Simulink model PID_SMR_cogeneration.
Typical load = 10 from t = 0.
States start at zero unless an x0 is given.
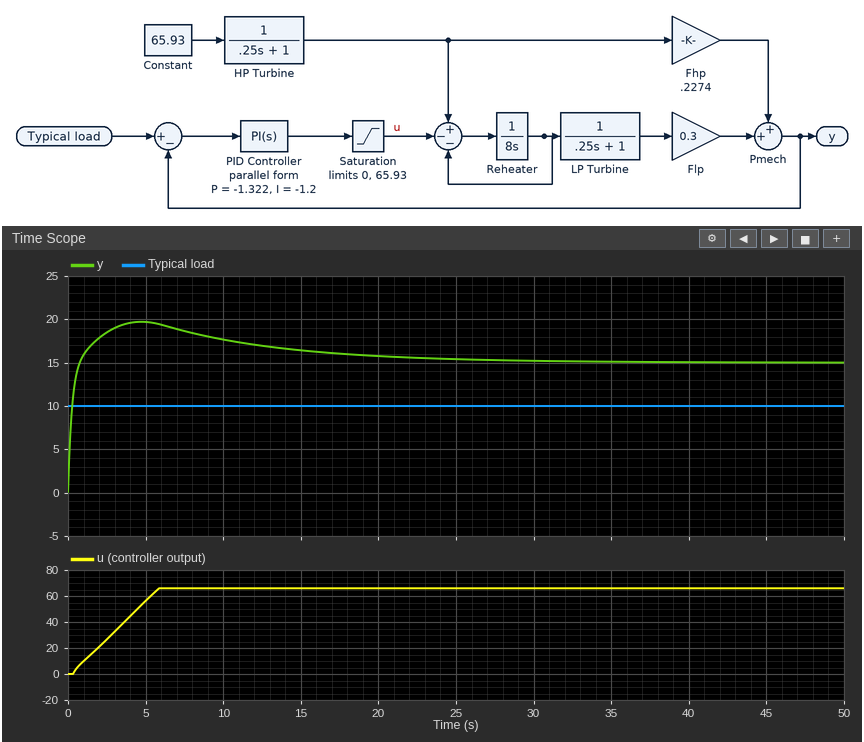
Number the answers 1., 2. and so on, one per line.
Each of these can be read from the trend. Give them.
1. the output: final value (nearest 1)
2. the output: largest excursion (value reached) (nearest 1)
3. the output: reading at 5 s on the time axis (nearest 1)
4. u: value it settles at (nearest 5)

1. 15
2. 20
3. 20
4. 65
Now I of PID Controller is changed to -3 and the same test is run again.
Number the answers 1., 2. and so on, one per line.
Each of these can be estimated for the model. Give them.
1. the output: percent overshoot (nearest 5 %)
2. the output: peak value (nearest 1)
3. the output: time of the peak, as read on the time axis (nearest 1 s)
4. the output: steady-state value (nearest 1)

1. 20 %
2. 18
3. 3 s
4. 15
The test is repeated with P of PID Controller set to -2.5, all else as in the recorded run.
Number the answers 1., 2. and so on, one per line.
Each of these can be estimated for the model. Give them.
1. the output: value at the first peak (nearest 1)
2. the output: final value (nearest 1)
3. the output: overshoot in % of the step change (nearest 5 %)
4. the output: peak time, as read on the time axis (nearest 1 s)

1. 19
2. 15
3. 25 %
4. 4 s
